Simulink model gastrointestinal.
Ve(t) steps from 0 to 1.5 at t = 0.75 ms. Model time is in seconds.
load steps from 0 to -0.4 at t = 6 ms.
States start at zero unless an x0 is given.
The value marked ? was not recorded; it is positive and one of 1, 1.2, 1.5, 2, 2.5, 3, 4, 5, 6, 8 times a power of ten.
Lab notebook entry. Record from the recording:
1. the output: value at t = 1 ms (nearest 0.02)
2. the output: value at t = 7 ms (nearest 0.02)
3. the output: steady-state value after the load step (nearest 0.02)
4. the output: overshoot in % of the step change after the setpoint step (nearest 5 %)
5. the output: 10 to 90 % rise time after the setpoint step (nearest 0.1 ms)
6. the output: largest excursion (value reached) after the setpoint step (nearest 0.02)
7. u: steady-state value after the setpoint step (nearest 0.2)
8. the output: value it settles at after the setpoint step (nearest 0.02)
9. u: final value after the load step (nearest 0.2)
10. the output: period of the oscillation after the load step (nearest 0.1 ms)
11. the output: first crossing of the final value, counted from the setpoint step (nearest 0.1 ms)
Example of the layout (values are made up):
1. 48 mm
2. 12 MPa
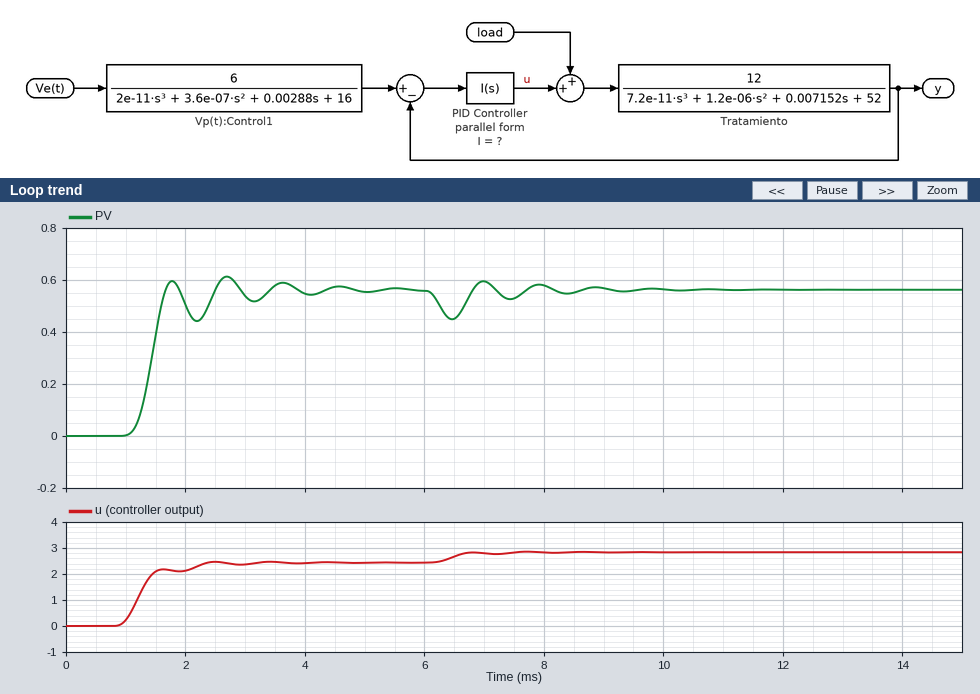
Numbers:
1. 0.00
2. 0.60
3. 0.56
4. 10 %
5. 0.4 ms
6. 0.62
7. 2.4
8. 0.56
9. 2.8
10. 1.0 ms
11. 0.9 ms
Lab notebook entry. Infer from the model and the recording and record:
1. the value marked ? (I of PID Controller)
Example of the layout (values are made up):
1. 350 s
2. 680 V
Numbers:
1. 8000
